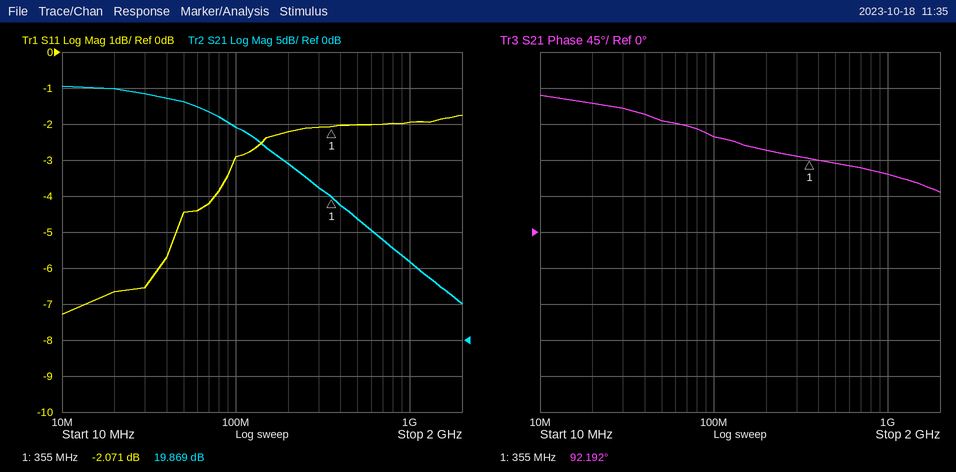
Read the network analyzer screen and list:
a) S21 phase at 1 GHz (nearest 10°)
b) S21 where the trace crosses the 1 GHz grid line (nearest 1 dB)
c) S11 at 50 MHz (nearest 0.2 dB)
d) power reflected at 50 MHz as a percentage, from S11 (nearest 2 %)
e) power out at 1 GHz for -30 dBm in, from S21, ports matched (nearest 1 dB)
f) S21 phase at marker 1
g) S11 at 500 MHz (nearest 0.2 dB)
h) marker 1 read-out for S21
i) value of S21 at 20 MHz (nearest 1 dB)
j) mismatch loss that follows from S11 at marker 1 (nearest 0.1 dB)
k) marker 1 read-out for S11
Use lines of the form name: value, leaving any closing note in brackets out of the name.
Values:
S21 phase at 1 GHz: 70°
S21 where the trace crosses the 1 GHz grid line: 11 dB
S11 at 50 MHz: -4.4 dB
power reflected at 50 MHz as a percentage, from S11: 36 %
power out at 1 GHz for -30 dBm in, from S21, ports matched: -19 dBm
S21 phase at marker 1: 92.192°
S11 at 500 MHz: -2.0 dB
marker 1 read-out for S21: 19.869 dB
value of S21 at 20 MHz: 35 dB
mismatch loss that follows from S11 at marker 1: 4.2 dB
marker 1 read-out for S11: -2.071 dB
